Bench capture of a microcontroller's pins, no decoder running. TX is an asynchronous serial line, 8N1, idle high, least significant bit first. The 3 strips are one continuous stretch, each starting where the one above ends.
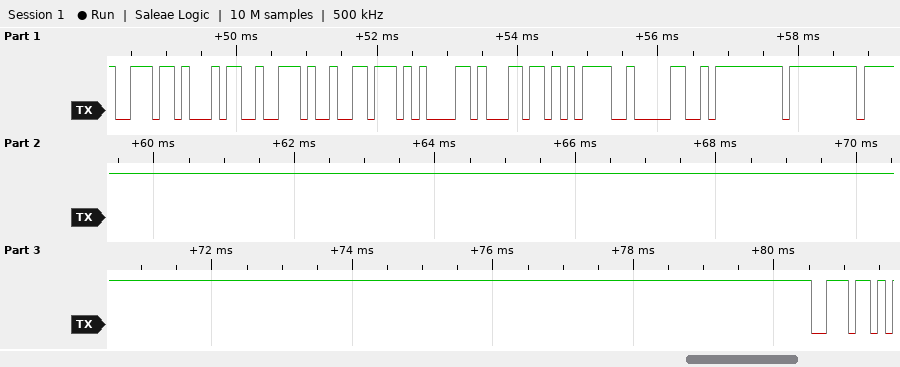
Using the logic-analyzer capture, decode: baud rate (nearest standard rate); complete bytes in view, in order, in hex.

9600 baud
0x6E 0x34 0x2E 0x76 0x61 0x6C 0x3D 0x30 0xFF 0xFF 0xFF 0x6E
